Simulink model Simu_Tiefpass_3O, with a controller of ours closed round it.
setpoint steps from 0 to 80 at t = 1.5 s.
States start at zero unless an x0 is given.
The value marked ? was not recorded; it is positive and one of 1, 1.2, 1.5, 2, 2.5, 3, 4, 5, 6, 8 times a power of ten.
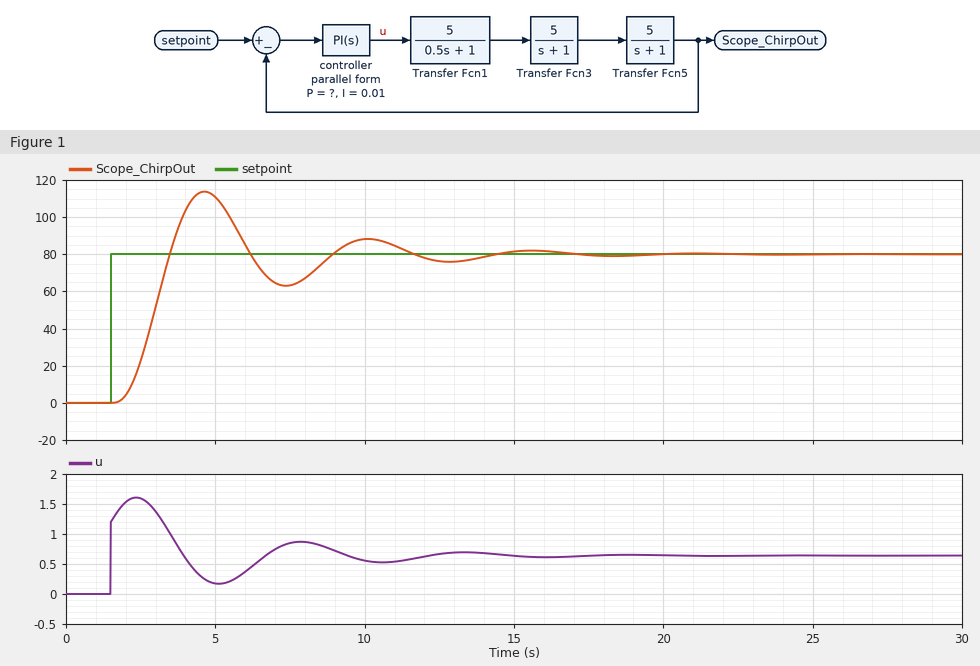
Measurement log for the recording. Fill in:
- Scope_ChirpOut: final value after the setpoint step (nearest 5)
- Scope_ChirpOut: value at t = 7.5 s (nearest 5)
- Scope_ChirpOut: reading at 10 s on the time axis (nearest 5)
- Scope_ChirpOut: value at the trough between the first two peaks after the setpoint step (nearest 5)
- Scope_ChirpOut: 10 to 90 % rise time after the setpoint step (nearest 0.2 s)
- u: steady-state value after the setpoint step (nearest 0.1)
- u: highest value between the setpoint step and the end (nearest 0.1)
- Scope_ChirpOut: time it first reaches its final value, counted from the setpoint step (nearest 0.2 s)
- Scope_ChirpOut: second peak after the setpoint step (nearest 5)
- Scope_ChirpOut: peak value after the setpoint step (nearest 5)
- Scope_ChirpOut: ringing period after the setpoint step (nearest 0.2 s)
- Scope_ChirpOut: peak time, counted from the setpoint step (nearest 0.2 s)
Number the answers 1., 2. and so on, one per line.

1. 80
2. 65
3. 90
4. 65
5. 1.2 s
6. 0.6
7. 1.6
8. 2.0 s
9. 90
10. 115
11. 5.4 s
12. 3.2 s
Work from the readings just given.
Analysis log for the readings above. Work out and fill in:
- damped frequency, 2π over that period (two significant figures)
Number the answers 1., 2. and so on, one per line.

1. 1.2 rad/s
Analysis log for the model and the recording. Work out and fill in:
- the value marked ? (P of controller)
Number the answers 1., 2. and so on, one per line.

1. 0.015
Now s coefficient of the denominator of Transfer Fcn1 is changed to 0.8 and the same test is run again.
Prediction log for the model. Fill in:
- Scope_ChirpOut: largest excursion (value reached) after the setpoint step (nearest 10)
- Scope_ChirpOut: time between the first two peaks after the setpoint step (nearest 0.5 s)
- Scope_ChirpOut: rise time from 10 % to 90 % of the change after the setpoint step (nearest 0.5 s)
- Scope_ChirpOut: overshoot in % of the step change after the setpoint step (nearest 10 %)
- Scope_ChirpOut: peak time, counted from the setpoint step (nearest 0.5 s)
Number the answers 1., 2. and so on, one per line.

1. 120
2. 6.0 s
3. 1.5 s
4. 50 %
5. 3.5 s
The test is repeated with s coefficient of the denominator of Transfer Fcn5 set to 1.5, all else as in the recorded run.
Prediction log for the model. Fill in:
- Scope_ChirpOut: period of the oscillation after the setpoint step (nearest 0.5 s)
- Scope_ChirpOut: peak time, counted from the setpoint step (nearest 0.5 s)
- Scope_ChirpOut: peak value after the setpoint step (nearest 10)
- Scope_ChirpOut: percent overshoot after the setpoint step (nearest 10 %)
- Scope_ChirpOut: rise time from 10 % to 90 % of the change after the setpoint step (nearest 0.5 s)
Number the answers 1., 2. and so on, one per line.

1. 6.5 s
2. 3.5 s
3. 120
4. 50 %
5. 1.5 s
